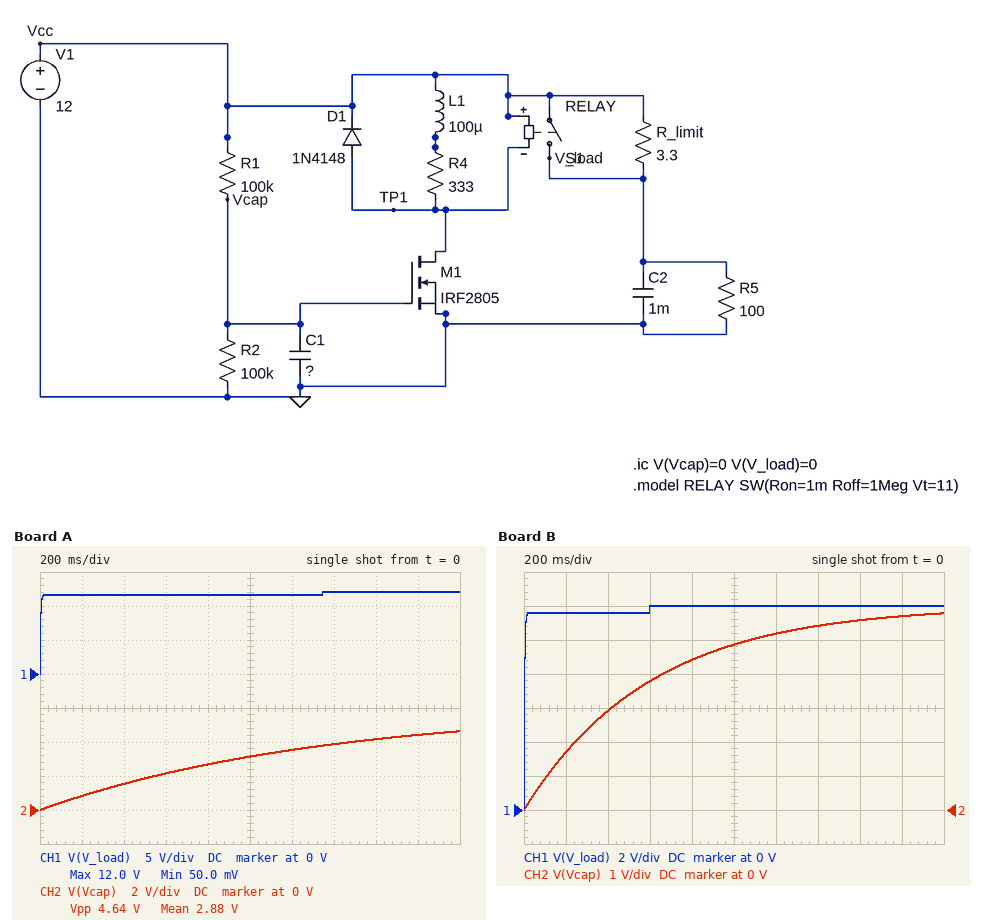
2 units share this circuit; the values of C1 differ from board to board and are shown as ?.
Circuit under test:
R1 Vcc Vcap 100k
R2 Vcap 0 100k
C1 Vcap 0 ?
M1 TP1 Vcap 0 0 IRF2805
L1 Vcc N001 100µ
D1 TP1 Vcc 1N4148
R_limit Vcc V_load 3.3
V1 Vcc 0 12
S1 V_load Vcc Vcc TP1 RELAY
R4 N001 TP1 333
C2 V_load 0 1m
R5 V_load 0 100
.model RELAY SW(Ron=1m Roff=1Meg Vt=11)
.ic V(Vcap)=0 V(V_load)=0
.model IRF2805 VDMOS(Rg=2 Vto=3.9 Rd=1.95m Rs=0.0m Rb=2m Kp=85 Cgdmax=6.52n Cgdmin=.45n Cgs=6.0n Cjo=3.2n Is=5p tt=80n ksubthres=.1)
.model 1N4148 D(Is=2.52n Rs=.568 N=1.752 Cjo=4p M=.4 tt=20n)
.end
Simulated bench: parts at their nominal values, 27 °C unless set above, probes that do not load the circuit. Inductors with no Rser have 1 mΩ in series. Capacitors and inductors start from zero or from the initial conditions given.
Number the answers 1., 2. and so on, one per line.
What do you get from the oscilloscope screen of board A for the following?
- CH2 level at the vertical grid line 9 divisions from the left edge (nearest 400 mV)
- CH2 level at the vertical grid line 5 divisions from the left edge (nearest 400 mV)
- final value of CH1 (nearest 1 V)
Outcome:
1. 4.4 V
2. 3.2 V
3. 12 V
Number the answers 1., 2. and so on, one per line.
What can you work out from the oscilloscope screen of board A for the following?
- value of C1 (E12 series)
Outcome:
1. 27 µF
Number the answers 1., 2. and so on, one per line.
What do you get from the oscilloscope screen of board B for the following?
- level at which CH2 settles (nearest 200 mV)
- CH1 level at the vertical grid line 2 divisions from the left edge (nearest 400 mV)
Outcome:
1. 5.8 V
2. 11.6 V
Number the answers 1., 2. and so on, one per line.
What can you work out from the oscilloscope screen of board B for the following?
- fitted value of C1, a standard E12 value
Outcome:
1. 12 µF
